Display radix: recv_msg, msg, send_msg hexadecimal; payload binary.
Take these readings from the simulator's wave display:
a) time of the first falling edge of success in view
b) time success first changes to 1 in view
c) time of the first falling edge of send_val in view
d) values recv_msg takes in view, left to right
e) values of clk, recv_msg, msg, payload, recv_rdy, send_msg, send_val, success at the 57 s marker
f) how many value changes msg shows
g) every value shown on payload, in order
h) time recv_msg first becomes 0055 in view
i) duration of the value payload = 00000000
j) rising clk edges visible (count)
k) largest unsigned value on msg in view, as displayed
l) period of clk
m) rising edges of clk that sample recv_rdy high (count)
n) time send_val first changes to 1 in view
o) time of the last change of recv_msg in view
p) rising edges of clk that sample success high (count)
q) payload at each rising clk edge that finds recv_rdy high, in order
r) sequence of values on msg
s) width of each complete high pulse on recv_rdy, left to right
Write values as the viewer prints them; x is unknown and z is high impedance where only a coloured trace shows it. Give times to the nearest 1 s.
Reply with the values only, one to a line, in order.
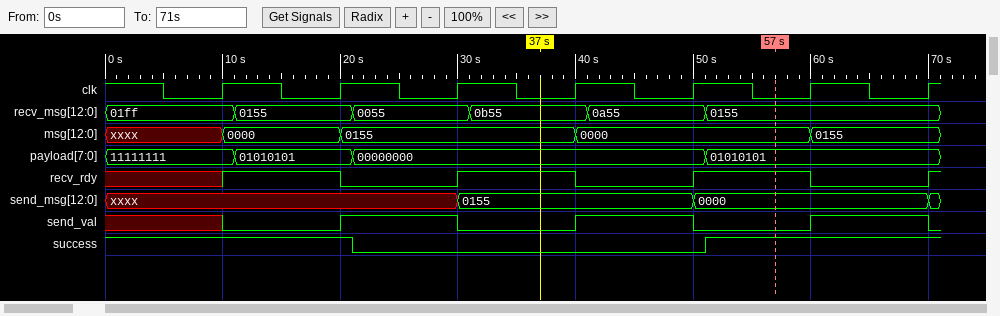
21 s
51 s
30 s
01ff, 0155, 0055, 0b55, 0a55, 0155
clk=0, recv_msg=0155, msg=0000, payload=01010101, recv_rdy=1, send_msg=0000, send_val=0, success=1
4
11111111, 01010101, 00000000, 01010101
21 s
30 s
7
0155
10 s
3
20 s
51 s
4
01010101, 00000000, 01010101
xxxx, 0000, 0155, 0000, 0155
10 s, 10 s
